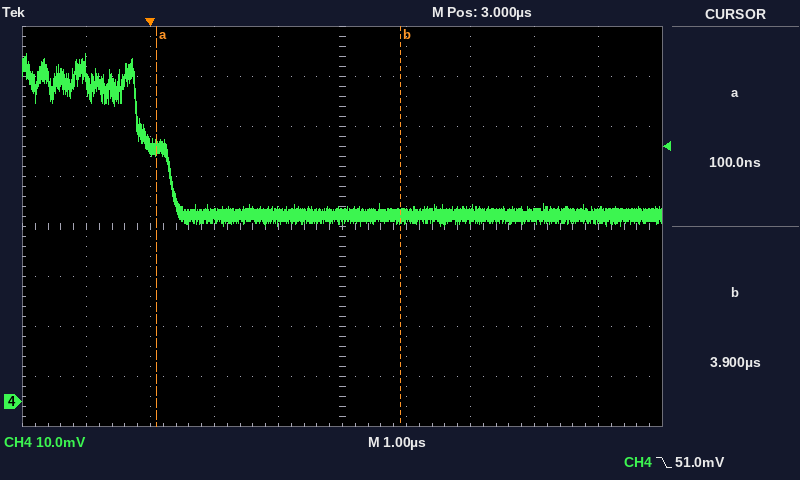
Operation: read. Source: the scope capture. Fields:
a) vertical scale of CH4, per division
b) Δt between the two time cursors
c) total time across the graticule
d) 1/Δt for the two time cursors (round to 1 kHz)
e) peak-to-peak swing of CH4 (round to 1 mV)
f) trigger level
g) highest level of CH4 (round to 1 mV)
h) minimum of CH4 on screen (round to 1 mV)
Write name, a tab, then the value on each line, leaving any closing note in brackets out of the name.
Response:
vertical scale of CH4, per division	10 mV
Δt between the two time cursors	3.8 µs
total time across the graticule	10 µs
1/Δt for the two time cursors	263 kHz
peak-to-peak swing of CH4	35 mV
trigger level	51.0 mV
highest level of CH4	70 mV
minimum of CH4 on screen	35 mV
